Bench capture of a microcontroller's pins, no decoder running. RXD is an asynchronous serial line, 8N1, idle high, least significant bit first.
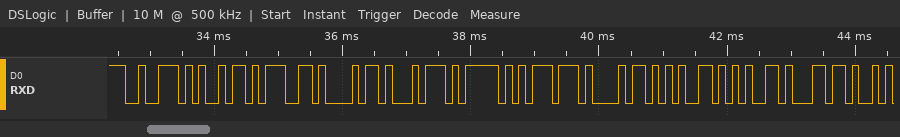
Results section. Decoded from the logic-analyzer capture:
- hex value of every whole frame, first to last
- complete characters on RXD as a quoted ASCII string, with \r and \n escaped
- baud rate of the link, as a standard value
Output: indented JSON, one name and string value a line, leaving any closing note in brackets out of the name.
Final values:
{
  "hex value of every whole frame, first to last": "72 69 67 68 74 5F 77 68 65 65 6C",
  "complete characters on RXD as a quoted ASCII string, with \\r and \\n escaped": "\"right_wheel\"",
  "baud rate of the link, as a standard value": "9600 baud"
}
